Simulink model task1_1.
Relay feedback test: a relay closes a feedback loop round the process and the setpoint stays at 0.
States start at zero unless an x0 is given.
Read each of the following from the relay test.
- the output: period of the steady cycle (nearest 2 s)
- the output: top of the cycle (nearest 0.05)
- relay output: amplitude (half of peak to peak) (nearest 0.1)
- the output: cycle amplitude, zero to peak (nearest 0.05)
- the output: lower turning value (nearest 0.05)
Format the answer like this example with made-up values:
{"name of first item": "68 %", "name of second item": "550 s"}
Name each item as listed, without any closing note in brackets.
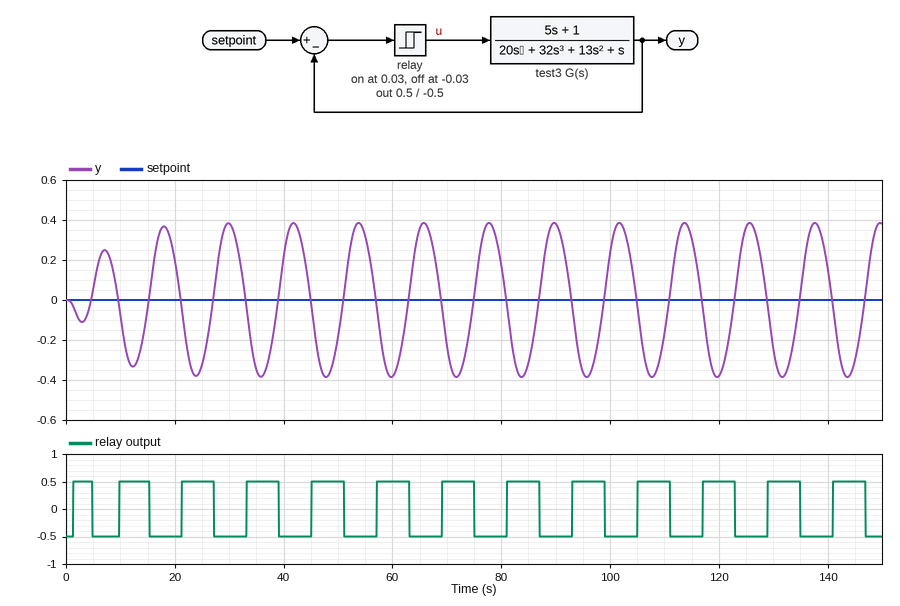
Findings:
{"the output: period of the steady cycle": "12 s", "the output: top of the cycle": "0.40", "relay output: amplitude (half of peak to peak)": "0.5", "the output: cycle amplitude, zero to peak": "0.40", "the output: lower turning value": "-0.40"}
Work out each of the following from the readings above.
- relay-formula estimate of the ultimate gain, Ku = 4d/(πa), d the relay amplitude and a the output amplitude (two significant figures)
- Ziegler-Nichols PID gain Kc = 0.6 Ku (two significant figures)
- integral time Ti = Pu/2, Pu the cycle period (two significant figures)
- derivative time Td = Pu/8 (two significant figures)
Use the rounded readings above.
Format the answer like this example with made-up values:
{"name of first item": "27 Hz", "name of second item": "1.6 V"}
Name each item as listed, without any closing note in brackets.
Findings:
{"relay-formula estimate of the ultimate gain, Ku = 4d/(πa), d the relay amplitude and a the output amplitude": "1.6", "Ziegler-Nichols PID gain Kc = 0.6 Ku": "0.96", "integral time Ti = Pu/2, Pu the cycle period": "6.0 s", "derivative time Td = Pu/8": "1.5 s"}
